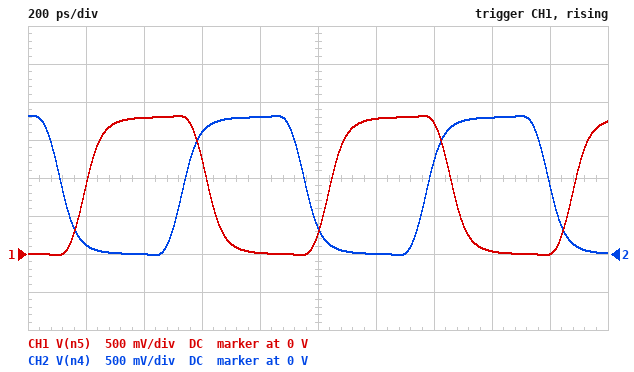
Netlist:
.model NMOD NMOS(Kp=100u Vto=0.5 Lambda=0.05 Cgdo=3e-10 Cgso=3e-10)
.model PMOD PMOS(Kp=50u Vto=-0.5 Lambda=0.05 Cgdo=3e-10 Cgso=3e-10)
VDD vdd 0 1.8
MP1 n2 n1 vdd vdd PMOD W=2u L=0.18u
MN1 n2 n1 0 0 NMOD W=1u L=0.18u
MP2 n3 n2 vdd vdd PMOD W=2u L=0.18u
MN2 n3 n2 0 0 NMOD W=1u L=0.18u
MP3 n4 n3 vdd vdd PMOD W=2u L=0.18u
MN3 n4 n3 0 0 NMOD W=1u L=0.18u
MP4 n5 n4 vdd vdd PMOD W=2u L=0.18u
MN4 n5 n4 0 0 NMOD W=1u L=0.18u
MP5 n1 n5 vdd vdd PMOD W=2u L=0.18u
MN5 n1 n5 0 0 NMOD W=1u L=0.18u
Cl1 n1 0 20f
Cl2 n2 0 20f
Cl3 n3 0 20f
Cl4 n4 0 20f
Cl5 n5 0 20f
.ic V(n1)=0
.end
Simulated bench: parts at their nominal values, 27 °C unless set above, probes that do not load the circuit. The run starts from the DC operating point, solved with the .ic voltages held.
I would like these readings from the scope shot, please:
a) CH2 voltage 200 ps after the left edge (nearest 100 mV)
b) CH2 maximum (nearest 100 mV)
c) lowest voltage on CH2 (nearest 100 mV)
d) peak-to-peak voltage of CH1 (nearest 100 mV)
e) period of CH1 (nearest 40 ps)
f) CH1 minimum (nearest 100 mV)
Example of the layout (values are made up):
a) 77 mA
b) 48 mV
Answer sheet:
a) 100 mV
b) 1.8 V
c) 0 V
d) 1.8 V
e) 840 ps
f) 0 V
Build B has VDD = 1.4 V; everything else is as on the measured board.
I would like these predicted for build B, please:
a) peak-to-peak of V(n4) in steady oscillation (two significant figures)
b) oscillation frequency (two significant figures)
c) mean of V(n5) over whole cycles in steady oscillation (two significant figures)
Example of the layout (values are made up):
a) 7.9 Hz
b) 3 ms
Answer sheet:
a) 1.4 V
b) 710 MHz
c) 700 mV
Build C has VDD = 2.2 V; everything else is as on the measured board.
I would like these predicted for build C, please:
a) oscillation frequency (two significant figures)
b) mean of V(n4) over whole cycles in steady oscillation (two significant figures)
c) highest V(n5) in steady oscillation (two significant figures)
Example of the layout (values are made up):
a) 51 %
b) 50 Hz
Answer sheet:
a) 1.7 GHz
b) 1.1 V
c) 2.2 V
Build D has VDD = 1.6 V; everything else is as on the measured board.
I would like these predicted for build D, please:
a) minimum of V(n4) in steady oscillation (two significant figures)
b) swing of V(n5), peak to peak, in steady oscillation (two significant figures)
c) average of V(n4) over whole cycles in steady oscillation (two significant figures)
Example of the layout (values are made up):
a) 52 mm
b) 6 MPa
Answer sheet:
a) -15 mV
b) 1.6 V
c) 800 mV
